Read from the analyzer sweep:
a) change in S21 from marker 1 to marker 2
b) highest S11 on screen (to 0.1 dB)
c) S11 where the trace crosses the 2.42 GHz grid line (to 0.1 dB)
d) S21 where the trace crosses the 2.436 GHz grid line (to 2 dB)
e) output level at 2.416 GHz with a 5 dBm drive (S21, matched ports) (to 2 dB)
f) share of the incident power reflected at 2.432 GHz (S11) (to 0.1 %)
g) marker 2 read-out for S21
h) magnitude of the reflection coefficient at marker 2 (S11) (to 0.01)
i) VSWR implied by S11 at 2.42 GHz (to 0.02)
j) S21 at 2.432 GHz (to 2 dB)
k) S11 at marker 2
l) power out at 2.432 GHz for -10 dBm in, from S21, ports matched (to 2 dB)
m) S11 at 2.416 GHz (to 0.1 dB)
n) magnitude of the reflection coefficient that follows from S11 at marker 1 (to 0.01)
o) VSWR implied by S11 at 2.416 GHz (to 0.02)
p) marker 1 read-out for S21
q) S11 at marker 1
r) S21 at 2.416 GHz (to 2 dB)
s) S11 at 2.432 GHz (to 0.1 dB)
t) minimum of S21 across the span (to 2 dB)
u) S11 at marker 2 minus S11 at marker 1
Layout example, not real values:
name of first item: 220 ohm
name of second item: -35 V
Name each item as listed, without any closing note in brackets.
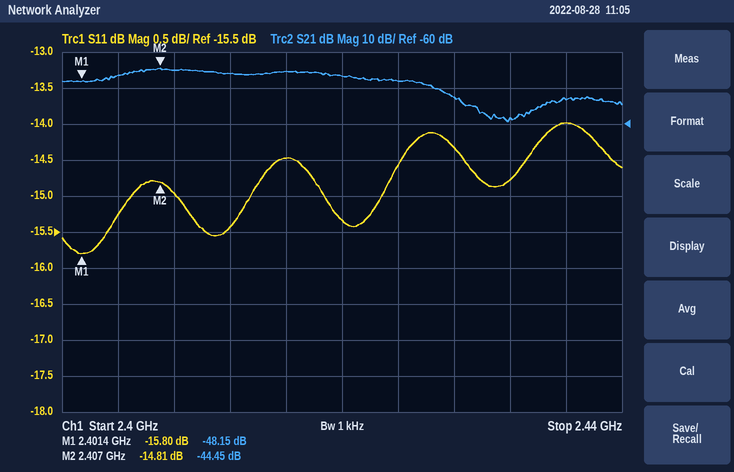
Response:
change in S21 from marker 1 to marker 2: 3.70 dB
highest S11 on screen: -14.0 dB
S11 where the trace crosses the 2.42 GHz grid line: -15.3 dB
S21 where the trace crosses the 2.436 GHz grid line: -54 dB
output level at 2.416 GHz with a 5 dBm drive (S21, matched ports): -40 dBm
share of the incident power reflected at 2.432 GHz (S11): 3.3 %
marker 2 read-out for S21: -44.45 dB
magnitude of the reflection coefficient at marker 2 (S11): 0.18
VSWR implied by S11 at 2.42 GHz: 1.42
S21 at 2.432 GHz: -58 dB
S11 at marker 2: -14.81 dB
power out at 2.432 GHz for -10 dBm in, from S21, ports matched: -68 dBm
S11 at 2.416 GHz: -14.5 dB
magnitude of the reflection coefficient that follows from S11 at marker 1: 0.16
VSWR implied by S11 at 2.416 GHz: 1.46
marker 1 read-out for S21: -48.15 dB
S11 at marker 1: -15.80 dB
S21 at 2.416 GHz: -46 dB
S11 at 2.432 GHz: -14.8 dB
minimum of S21 across the span: -60 dB
S11 at marker 2 minus S11 at marker 1: 0.99 dB
